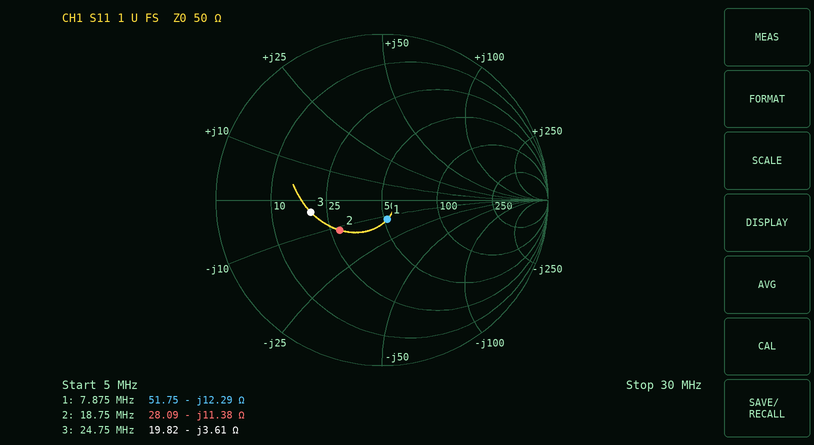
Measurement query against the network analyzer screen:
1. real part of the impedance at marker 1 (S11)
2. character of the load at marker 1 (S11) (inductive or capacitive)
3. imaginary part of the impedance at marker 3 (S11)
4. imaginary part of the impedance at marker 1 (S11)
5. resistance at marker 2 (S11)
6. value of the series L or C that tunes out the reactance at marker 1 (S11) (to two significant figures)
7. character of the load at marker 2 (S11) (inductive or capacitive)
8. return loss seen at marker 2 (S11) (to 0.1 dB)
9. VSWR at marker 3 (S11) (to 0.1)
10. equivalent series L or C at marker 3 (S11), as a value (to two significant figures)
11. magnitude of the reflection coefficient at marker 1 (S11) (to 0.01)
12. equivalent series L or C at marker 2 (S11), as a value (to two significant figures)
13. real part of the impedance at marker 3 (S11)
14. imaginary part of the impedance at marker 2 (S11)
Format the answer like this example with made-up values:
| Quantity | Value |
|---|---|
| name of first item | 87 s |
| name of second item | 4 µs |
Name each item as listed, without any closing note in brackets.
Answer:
| Quantity | Value |
|---|---|
| real part of the impedance at marker 1 | 51.75 Ω |
| character of the load at marker 1 (S11) | capacitive |
| imaginary part of the impedance at marker 3 | -3.61 Ω |
| imaginary part of the impedance at marker 1 | -12.29 Ω |
| resistance at marker 2 | 28.09 Ω |
| value of the series L or C that tunes out the reactance at marker 1 (S11) | 250 nH |
| character of the load at marker 2 (S11) | capacitive |
| return loss seen at marker 2 (S11) | 10.1 dB |
| VSWR at marker 3 (S11) | 2.5 |
| equivalent series L or C at marker 3 (S11), as a value | 1.8 nF |
| magnitude of the reflection coefficient at marker 1 (S11) | 0.12 |
| equivalent series L or C at marker 2 (S11), as a value | 750 pF |
| real part of the impedance at marker 3 | 19.82 Ω |
| imaginary part of the impedance at marker 2 | -11.38 Ω |
